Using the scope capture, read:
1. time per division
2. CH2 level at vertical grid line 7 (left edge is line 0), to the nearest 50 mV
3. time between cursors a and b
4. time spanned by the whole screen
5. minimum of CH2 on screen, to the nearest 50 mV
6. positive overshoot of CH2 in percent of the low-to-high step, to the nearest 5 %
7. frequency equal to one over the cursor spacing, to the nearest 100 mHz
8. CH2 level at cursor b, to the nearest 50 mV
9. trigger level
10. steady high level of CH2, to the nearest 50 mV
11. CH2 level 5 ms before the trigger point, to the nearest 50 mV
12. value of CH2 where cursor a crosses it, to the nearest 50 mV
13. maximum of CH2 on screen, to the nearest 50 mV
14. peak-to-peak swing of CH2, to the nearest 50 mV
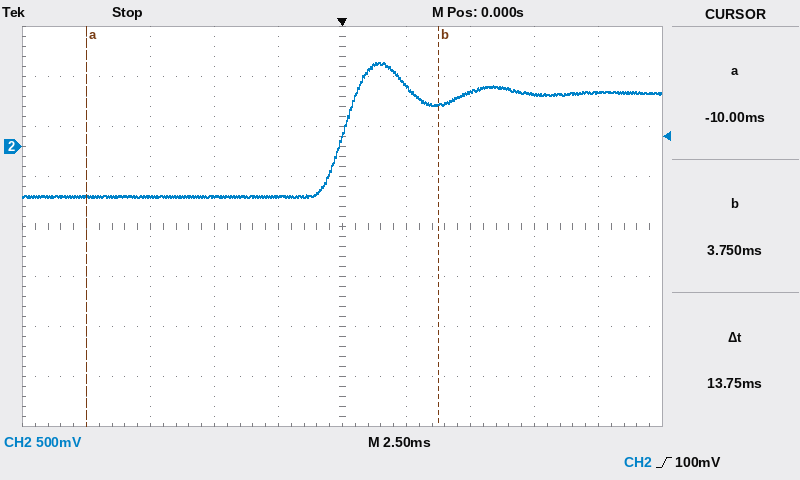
2.5 ms
550 mV
13.75 ms
25 ms
-500 mV
30 %
72.7 Hz
400 mV
100 mV
550 mV
-500 mV
-500 mV
850 mV
1.35 V
